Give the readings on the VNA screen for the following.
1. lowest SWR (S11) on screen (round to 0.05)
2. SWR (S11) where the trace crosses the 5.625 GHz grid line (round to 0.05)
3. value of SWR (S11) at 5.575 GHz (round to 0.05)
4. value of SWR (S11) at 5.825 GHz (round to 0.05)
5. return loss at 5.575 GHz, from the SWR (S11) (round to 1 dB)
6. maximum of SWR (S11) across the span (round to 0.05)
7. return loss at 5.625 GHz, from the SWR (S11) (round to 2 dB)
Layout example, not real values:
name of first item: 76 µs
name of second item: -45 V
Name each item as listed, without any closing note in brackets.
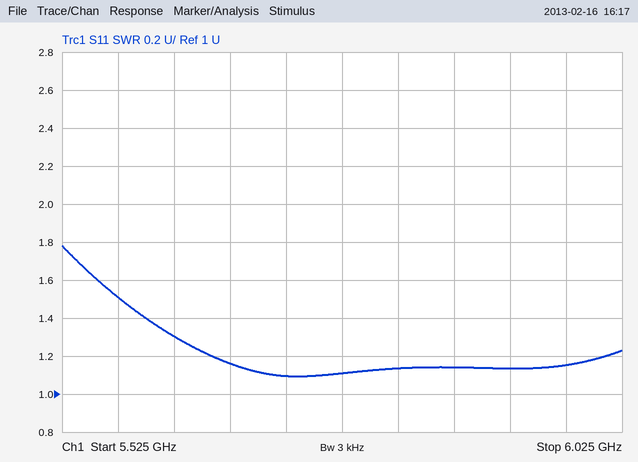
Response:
lowest SWR (S11) on screen: 1.10
SWR (S11) where the trace crosses the 5.625 GHz grid line: 1.30
value of SWR (S11) at 5.575 GHz: 1.50
value of SWR (S11) at 5.825 GHz: 1.15
return loss at 5.575 GHz, from the SWR (S11): 14 dB
maximum of SWR (S11) across the span: 1.80
return loss at 5.625 GHz, from the SWR (S11): 18 dB
